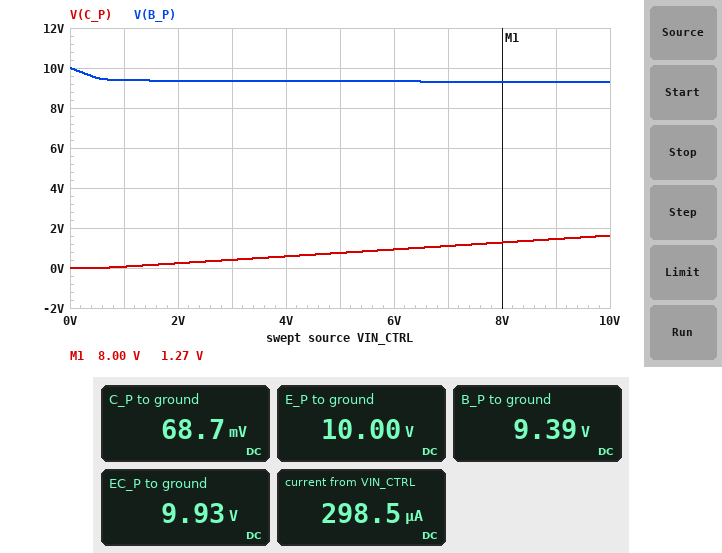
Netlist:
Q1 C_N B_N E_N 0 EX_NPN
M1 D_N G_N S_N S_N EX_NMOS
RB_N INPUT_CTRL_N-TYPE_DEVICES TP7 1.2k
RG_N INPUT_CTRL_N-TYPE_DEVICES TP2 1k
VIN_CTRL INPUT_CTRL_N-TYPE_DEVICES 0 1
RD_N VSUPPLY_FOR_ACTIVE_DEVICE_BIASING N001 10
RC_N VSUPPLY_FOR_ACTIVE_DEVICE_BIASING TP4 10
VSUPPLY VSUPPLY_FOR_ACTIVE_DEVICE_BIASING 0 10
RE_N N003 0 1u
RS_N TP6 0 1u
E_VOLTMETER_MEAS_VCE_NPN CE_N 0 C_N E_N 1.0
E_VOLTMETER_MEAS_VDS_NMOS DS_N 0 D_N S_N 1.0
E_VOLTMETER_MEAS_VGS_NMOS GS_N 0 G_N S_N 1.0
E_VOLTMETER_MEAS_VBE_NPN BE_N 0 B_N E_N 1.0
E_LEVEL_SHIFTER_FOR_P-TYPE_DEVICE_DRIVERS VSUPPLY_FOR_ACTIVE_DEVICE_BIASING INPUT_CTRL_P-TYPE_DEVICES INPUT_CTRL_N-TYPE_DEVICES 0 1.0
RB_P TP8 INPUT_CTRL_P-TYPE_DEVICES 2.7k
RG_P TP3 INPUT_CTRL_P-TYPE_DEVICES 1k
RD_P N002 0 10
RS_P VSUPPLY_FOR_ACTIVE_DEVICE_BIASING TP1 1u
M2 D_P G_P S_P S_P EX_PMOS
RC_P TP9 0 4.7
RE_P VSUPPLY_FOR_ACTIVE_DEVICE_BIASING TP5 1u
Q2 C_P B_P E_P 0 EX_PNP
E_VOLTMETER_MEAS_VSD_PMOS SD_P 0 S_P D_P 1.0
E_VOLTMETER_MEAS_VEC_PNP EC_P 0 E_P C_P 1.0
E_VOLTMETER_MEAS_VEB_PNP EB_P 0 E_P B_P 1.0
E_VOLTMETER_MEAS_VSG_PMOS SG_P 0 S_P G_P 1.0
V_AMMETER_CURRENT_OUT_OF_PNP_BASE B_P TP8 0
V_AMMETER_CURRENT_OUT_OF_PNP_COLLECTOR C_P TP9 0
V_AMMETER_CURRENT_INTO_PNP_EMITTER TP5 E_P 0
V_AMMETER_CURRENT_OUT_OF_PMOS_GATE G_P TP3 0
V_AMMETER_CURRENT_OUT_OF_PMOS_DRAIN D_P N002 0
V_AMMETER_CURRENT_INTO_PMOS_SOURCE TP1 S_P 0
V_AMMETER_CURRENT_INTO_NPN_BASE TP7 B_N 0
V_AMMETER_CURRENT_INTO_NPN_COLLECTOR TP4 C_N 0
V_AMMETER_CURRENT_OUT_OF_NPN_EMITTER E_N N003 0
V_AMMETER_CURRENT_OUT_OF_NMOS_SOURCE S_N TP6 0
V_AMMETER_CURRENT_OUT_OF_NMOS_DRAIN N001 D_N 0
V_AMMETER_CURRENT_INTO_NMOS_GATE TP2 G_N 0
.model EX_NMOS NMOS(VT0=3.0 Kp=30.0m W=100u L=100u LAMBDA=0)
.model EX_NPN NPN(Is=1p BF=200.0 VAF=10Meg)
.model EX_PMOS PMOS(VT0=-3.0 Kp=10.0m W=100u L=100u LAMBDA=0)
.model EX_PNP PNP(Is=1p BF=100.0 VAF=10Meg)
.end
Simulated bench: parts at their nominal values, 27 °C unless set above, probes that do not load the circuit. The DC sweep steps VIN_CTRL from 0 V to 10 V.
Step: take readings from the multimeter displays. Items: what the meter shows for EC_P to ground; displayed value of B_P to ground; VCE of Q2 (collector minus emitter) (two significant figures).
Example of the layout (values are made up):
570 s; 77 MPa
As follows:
9.93 V; 9.39 V; -9.9 V
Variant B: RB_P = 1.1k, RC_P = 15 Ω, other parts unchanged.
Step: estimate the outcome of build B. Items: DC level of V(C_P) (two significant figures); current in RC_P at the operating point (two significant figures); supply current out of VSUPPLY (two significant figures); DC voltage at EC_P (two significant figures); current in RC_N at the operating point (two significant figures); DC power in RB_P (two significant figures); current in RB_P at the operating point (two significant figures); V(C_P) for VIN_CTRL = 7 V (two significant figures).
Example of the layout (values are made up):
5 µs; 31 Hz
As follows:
510 mV; 34 mA; 94 mA; 9.5 V; 60 mA; 130 µW; 340 µA; 8.6 V
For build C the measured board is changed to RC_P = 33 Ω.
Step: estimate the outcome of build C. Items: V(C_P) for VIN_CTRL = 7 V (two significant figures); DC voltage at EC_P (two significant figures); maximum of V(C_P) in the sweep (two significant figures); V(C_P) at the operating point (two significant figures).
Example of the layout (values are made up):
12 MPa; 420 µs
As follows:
7.7 V; 9.5 V; 9.8 V; 480 mV
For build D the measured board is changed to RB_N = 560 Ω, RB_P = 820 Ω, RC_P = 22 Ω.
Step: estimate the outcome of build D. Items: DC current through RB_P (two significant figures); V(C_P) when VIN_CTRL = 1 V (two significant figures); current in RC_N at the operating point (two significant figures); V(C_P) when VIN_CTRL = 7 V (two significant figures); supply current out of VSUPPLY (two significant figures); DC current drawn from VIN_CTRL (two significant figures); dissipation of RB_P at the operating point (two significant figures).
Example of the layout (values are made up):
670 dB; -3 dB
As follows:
450 µA; 980 mV; 120 mA; 9.9 V; 170 mA; 610 µA; 160 µW
